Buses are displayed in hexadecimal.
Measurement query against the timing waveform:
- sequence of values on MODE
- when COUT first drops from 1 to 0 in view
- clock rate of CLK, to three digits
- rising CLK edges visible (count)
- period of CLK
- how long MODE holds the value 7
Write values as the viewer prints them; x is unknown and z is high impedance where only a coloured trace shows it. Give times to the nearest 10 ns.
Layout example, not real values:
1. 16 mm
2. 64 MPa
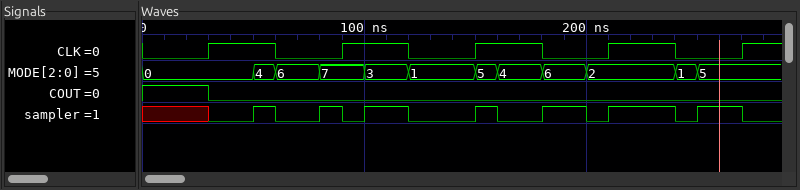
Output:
1. 0, 4, 6, 7, 3, 1, 5, 4, 6, 2, 1, 5
2. 30 ns
3. 16.7 MHz
4. 5
5. 60 ns
6. 20 ns
